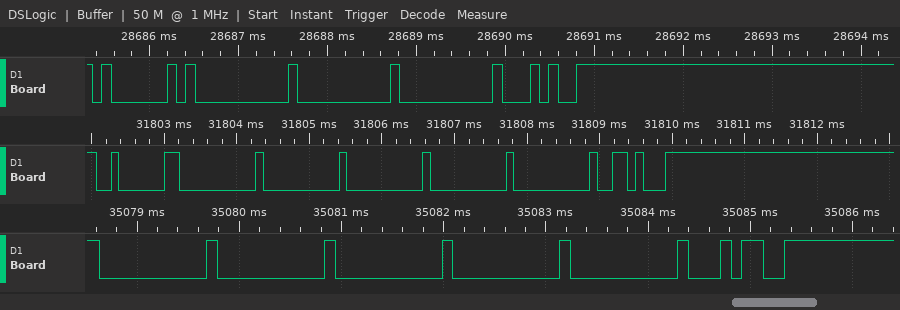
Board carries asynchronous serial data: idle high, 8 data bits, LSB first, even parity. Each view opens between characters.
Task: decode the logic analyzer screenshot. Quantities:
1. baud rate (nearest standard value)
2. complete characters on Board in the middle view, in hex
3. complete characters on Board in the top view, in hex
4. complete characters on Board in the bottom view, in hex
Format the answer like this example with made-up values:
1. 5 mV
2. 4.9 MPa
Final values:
1. 9600 baud
2. 02, 00, 00, 00, 00, 00, 16
3. 81, 00, 00, 00, 94
4. 00, 00, 00, 00, 00, 34
